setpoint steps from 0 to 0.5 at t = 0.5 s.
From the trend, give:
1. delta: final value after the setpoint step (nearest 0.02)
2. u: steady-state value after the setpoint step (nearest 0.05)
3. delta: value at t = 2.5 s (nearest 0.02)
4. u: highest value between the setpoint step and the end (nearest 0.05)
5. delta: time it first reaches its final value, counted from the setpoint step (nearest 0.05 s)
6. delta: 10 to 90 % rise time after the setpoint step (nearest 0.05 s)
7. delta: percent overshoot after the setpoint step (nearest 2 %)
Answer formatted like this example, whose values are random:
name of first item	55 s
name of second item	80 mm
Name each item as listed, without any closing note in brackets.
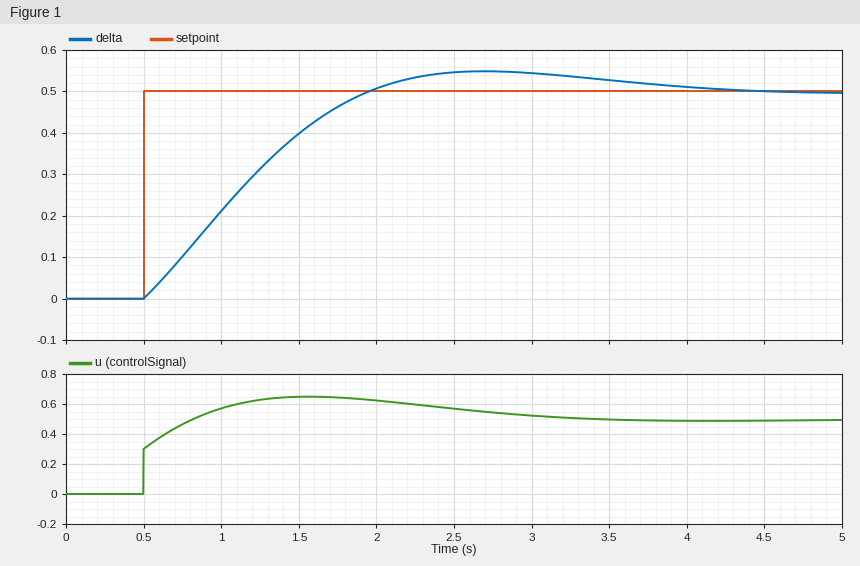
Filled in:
delta: final value after the setpoint step	0.50
u: steady-state value after the setpoint step	0.50
delta: value at t = 2.5 s	0.54
u: highest value between the setpoint step and the end	0.65
delta: time it first reaches its final value, counted from the setpoint step	1.45 s
delta: 10 to 90 % rise time after the setpoint step	1.05 s
delta: percent overshoot after the setpoint step	10 %
